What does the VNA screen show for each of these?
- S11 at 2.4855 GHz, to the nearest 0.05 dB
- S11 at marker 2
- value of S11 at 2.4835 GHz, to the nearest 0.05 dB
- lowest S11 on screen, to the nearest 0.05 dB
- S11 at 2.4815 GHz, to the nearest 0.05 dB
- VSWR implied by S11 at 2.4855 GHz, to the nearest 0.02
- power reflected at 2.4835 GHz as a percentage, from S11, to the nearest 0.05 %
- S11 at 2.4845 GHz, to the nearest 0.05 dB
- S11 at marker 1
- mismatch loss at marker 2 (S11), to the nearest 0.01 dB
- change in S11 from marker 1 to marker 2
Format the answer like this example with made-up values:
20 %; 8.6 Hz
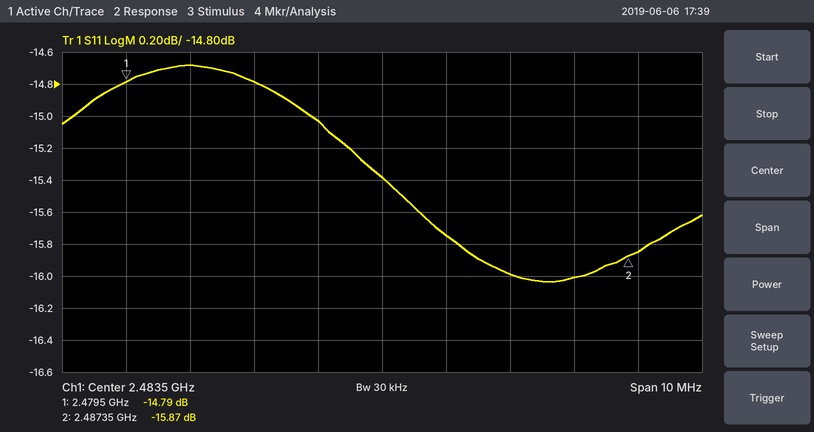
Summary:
-16.00 dB; -15.87 dB; -15.40 dB; -16.05 dB; -14.80 dB; 1.38; 2.90 %; -15.75 dB; -14.79 dB; 0.11 dB; -1.08 dB
